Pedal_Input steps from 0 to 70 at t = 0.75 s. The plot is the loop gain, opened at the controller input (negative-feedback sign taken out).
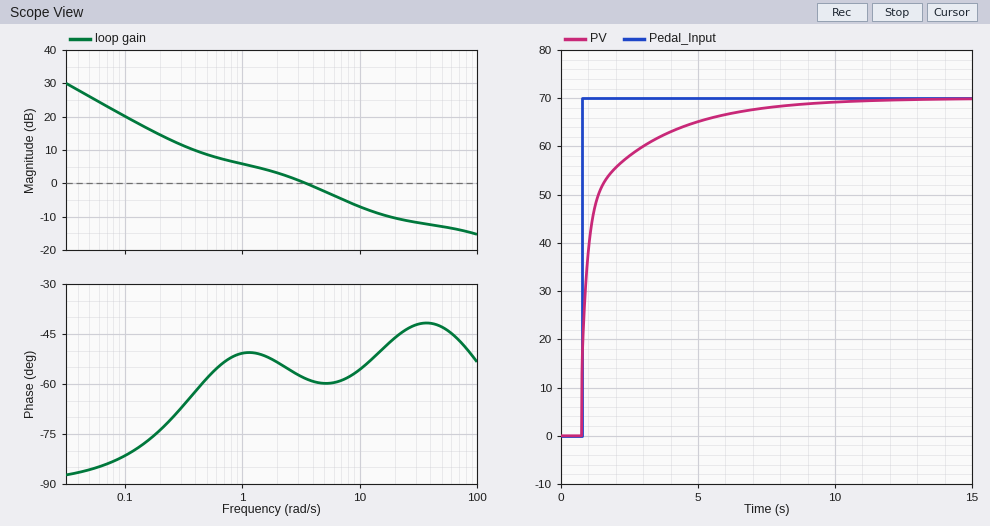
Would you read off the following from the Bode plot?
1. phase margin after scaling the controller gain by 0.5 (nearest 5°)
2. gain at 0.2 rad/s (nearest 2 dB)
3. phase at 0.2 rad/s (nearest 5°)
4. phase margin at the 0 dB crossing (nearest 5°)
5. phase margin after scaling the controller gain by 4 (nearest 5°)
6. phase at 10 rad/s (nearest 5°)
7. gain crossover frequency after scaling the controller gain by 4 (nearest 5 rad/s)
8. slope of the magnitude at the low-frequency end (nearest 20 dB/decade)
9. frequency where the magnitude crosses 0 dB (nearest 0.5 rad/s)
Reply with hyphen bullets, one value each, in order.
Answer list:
- 130°
- 14 dB
- -75°
- 120°
- 140°
- -55°
- 35 rad/s
- -20 dB/decade
- 3.5 rad/s
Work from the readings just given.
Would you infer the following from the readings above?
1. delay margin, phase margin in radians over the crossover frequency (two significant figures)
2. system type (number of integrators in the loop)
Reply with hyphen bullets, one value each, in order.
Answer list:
- 0.60 s
- 1
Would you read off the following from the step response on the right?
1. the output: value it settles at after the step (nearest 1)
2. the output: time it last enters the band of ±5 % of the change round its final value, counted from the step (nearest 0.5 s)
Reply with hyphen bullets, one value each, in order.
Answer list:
- 70
- 5.0 s
